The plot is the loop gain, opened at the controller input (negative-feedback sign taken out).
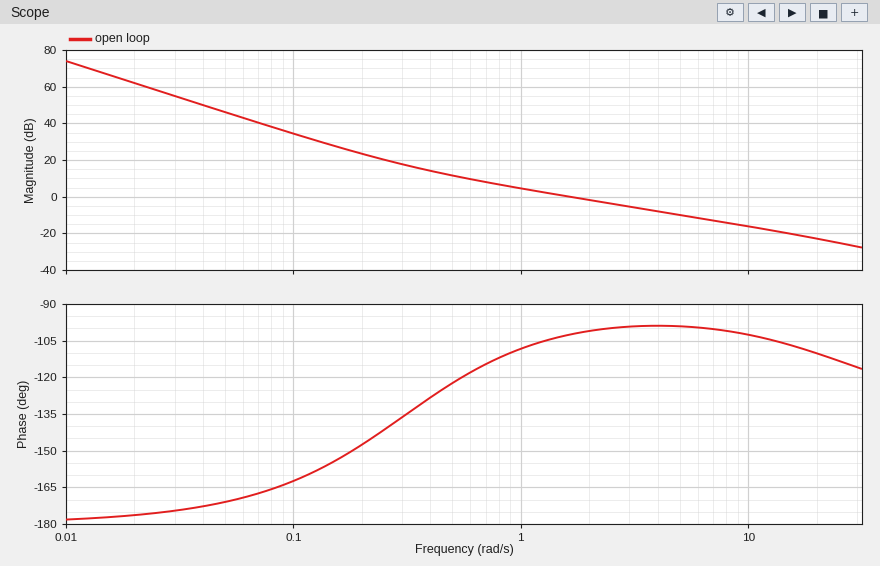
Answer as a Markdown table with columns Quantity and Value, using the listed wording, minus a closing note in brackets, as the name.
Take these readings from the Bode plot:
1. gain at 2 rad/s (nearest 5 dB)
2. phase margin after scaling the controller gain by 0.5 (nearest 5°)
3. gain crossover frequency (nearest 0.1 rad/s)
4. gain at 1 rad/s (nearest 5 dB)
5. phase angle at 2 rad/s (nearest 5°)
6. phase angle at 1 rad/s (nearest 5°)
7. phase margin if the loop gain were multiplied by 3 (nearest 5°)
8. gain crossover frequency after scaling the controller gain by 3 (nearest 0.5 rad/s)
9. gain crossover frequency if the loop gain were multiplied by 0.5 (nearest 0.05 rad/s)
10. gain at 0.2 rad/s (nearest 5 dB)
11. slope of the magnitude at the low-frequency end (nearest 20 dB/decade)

| Quantity | Value |
|---|---|
| gain at 2 rad/s | 0 dB |
| phase margin after scaling the controller gain by 0.5 | 70° |
| gain crossover frequency | 1.6 rad/s |
| gain at 1 rad/s | 5 dB |
| phase angle at 2 rad/s | -100° |
| phase angle at 1 rad/s | -110° |
| phase margin if the loop gain were multiplied by 3 | 80° |
| gain crossover frequency after scaling the controller gain by 3 | 5.0 rad/s |
| gain crossover frequency if the loop gain were multiplied by 0.5 | 0.85 rad/s |
| gain at 0.2 rad/s | 25 dB |
| slope of the magnitude at the low-frequency end | -40 dB/decade |
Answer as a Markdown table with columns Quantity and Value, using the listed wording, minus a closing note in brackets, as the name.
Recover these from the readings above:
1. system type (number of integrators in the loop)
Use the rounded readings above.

| Quantity | Value |
|---|---|
| system type | 2 |
